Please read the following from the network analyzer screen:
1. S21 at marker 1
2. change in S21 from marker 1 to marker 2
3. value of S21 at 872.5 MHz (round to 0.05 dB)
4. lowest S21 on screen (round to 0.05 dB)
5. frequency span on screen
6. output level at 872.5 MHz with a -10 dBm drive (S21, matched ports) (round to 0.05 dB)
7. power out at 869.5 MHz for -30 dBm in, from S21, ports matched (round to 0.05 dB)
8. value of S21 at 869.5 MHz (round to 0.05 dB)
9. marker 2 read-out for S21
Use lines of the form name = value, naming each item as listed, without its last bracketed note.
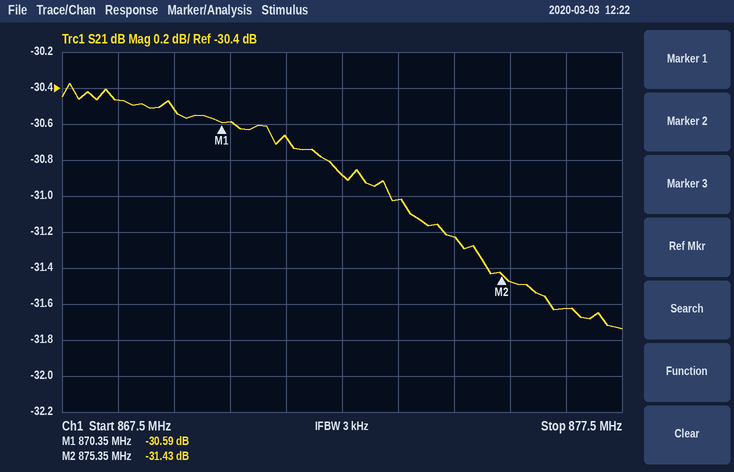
S21 at marker 1 = -30.59 dB
change in S21 from marker 1 to marker 2 = -0.84 dB
value of S21 at 872.5 MHz = -30.90 dB
lowest S21 on screen = -31.75 dB
frequency span on screen = 10 MHz
output level at 872.5 MHz with a -10 dBm drive (S21, matched ports) = -40.90 dBm
power out at 869.5 MHz for -30 dBm in, from S21, ports matched = -60.50 dBm
value of S21 at 869.5 MHz = -30.50 dB
marker 2 read-out for S21 = -31.43 dB
